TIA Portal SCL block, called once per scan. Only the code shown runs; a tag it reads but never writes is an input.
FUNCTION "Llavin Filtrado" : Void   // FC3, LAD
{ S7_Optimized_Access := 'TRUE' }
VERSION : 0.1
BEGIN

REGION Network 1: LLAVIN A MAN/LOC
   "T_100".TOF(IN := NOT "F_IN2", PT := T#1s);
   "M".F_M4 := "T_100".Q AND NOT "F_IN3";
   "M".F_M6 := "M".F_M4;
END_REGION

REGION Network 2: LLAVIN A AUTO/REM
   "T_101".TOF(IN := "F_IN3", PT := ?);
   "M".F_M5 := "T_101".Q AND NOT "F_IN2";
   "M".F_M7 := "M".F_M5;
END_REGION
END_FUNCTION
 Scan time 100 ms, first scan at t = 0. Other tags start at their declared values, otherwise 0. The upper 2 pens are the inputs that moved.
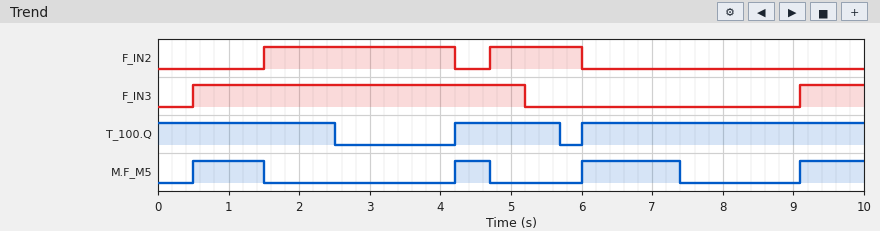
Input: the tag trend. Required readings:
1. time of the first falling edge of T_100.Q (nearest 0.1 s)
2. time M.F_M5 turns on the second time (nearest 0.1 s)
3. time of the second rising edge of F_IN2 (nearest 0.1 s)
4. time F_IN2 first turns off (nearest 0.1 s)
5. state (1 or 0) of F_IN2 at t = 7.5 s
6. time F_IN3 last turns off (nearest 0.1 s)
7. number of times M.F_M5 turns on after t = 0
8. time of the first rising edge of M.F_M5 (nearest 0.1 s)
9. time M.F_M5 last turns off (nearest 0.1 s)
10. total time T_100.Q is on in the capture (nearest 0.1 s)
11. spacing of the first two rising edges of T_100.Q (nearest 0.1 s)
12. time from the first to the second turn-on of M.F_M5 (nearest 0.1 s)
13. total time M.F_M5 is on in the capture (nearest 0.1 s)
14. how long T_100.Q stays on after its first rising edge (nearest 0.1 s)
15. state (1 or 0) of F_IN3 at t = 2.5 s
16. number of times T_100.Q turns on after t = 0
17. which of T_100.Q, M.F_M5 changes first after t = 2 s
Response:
2.5 s
4.2 s
4.7 s
4.2 s
0
5.2 s
4
0.5 s
7.4 s
8.0 s
1.8 s
3.7 s
3.8 s
1.5 s
1
2
T_100.Q
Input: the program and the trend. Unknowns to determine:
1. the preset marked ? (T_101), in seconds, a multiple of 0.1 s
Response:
2.2 s
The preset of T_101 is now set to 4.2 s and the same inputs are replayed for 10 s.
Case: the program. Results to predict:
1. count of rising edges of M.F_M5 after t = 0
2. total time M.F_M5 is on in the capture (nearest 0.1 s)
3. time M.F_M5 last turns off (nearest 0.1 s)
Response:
3
5.5 s
4.7 s
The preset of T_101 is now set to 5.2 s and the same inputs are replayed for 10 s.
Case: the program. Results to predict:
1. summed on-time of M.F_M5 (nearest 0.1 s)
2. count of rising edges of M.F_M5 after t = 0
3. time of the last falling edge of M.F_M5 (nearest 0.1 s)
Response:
5.5 s
3
4.7 s
